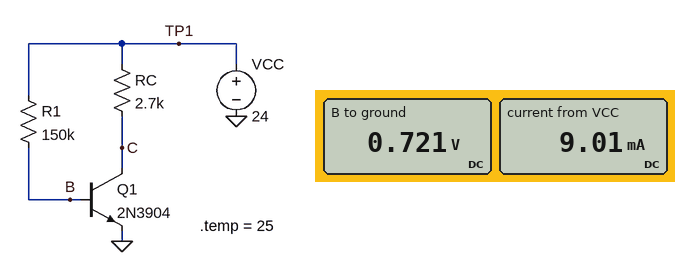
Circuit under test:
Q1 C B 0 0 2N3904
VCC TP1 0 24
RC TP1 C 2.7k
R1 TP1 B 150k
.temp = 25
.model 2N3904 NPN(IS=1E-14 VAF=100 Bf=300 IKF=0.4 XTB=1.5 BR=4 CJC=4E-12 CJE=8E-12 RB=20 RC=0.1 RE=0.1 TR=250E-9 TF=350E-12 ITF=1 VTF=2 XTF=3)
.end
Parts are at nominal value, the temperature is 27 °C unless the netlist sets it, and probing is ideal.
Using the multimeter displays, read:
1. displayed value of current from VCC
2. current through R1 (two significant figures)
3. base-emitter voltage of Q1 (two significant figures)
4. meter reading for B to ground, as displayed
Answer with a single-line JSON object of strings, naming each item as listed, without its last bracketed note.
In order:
{"displayed value of current from VCC": "9.01 mA", "current through R1": "160 µA", "base-emitter voltage of Q1": "720 mV", "meter reading for B to ground, as displayed": "0.721 V"}
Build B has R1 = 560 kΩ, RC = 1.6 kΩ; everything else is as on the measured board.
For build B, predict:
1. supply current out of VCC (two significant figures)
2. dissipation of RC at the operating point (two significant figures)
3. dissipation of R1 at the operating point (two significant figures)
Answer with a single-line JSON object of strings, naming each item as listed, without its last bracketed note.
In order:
{"supply current out of VCC": "12 mA", "dissipation of RC at the operating point": "250 mW", "dissipation of R1 at the operating point": "970 µW"}
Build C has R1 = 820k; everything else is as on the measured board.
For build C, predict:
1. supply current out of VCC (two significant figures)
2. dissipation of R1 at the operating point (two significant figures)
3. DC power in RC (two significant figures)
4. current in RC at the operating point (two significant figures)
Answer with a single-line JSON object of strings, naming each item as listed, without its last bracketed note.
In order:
{"supply current out of VCC": "8.4 mA", "dissipation of R1 at the operating point": "660 µW", "DC power in RC": "190 mW", "current in RC at the operating point": "8.3 mA"}
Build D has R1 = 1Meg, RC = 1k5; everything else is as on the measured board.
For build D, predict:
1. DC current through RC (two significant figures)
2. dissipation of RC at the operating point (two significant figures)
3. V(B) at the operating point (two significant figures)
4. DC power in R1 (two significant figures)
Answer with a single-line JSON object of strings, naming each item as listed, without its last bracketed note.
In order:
{"DC current through RC": "7.6 mA", "dissipation of RC at the operating point": "87 mW", "V(B) at the operating point": "710 mV", "DC power in R1": "540 µW"}
